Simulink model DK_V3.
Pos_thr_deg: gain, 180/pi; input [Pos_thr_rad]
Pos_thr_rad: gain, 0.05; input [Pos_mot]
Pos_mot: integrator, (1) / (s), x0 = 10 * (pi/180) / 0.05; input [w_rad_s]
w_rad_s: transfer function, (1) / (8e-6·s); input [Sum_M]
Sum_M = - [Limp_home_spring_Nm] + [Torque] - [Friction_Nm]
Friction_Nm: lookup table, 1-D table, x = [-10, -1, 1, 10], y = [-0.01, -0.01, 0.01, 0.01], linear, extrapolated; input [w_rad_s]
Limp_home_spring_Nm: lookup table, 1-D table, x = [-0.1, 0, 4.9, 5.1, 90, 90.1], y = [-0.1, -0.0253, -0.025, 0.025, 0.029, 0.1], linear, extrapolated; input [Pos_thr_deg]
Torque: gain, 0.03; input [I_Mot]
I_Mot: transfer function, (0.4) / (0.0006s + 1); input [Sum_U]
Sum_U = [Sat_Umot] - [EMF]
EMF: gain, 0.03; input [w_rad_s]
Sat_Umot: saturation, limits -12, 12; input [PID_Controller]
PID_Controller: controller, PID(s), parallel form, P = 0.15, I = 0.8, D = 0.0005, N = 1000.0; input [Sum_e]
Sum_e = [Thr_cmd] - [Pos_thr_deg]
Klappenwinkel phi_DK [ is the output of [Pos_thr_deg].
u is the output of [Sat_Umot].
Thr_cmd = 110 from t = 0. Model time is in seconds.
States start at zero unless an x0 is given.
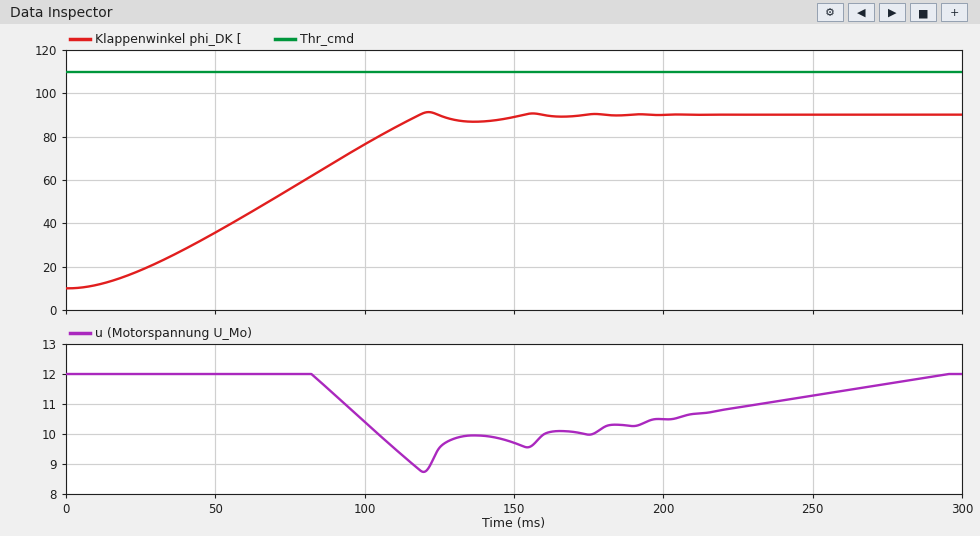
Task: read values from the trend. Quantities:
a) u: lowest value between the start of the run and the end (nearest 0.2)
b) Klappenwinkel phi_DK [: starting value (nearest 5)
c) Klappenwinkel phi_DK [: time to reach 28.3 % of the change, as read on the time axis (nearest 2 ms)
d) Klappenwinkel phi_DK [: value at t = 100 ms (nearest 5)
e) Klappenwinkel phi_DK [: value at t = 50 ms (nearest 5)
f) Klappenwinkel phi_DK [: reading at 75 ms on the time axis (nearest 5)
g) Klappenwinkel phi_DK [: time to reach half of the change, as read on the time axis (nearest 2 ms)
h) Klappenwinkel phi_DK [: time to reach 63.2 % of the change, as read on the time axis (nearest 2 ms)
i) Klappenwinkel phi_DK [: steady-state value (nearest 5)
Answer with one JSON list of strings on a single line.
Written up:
["8.8", "10", "46 ms", "75", "35", "55", "68 ms", "80 ms", "90"]
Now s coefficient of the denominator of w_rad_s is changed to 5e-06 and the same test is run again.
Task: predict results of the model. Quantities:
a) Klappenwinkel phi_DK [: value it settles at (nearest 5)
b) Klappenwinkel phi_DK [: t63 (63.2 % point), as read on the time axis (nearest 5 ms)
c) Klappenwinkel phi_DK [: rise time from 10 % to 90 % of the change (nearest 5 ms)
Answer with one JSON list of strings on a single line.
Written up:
["90", "75 ms", "80 ms"]
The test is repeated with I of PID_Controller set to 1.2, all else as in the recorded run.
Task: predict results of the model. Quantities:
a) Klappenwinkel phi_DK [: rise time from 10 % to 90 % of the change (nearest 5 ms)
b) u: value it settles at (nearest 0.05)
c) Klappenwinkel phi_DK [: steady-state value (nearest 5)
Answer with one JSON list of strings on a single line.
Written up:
["80 ms", "12.00", "90"]
